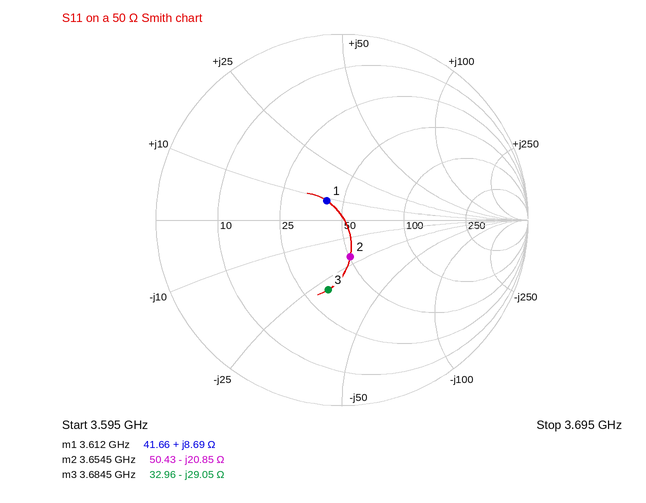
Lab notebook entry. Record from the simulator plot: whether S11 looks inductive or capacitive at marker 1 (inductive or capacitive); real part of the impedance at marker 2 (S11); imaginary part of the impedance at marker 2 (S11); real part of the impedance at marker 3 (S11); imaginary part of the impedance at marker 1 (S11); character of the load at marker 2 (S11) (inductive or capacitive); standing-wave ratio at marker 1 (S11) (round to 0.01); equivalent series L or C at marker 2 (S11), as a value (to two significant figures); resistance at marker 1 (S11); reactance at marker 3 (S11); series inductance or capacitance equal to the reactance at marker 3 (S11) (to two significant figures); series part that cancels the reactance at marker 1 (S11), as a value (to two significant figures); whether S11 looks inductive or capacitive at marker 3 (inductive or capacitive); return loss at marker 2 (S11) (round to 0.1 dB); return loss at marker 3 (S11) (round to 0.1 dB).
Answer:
inductive
50.43 Ω
-20.85 Ω
32.96 Ω
+8.69 Ω
capacitive
1.30
2.1 pF
41.66 Ω
-29.05 Ω
1.5 pF
5.1 pF
capacitive
13.8 dB
8.3 dB
